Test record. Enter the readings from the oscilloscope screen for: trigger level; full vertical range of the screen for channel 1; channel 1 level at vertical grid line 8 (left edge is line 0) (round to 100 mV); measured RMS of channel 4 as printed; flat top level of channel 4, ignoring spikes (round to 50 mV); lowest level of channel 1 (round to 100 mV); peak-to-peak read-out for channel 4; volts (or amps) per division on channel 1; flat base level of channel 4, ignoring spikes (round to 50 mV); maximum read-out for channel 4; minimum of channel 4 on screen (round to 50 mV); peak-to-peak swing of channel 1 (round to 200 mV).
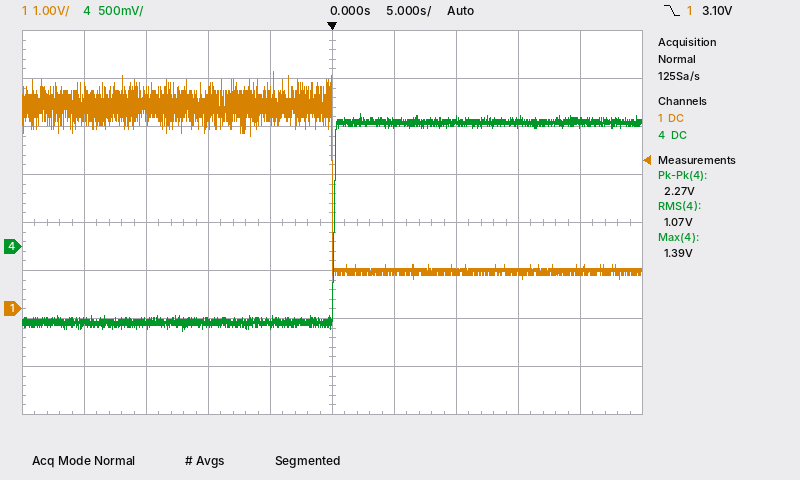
3.10 V
8 V
800 mV
1.07 V
1.30 V
600 mV
2.27 V
1 V
-800 mV
1.39 V
-900 mV
4.4 V
